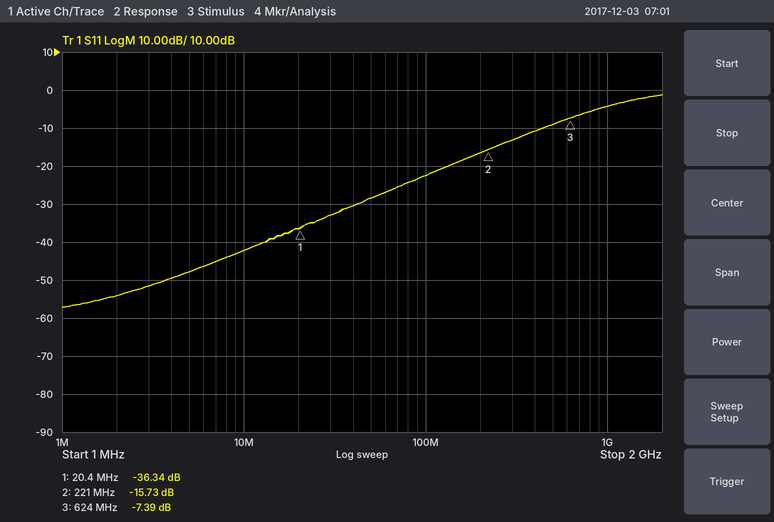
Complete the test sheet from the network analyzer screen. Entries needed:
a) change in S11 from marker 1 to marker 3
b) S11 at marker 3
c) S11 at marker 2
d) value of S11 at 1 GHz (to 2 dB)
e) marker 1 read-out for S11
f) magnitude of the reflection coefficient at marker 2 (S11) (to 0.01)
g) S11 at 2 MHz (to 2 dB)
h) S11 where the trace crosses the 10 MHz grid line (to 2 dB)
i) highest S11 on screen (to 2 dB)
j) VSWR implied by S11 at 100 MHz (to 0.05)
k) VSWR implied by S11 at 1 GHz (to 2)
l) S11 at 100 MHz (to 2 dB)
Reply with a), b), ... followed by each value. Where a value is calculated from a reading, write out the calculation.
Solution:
a) -7.39 − (-36.34) = 28.95 dB
b) -7.39 dB
c) -15.73 dB
d) -4 dB
e) -36.34 dB
f) 10^(-15.73/20) ≈ 0.16
g) -54 dB
h) -42 dB
i) -2 dB
j) |Γ| = 10^(-22/20) = 0.0794; VSWR = (1 + 0.0794)/(1 − 0.0794) ≈ 1.17, so 1.15 to the nearest 0.05
k) |Γ| = 10^(-4/20) = 0.6310; VSWR = (1 + 0.6310)/(1 − 0.6310) ≈ 4
l) -22 dB
